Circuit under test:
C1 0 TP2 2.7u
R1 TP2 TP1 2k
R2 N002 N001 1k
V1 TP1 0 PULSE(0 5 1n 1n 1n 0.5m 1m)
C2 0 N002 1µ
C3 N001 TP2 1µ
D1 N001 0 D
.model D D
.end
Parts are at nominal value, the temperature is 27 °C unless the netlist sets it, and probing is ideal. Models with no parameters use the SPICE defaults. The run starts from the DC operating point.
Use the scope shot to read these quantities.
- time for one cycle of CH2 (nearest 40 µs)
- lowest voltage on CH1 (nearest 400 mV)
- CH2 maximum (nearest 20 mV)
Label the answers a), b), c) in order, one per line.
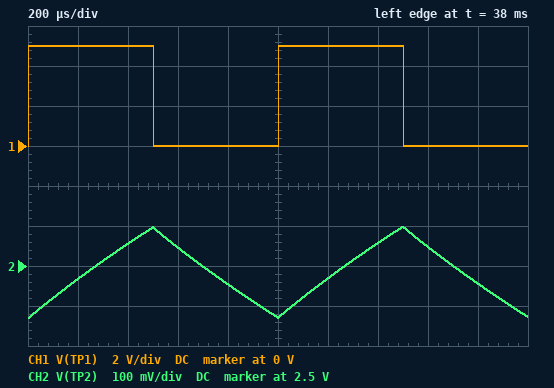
a) 1.00 ms
b) 0 V
c) 2.60 V
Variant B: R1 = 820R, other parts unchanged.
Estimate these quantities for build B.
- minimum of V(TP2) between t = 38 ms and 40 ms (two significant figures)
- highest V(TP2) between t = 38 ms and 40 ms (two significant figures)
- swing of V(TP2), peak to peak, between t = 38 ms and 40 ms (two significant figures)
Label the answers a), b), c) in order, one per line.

a) 2.2 V
b) 2.8 V
c) 550 mV
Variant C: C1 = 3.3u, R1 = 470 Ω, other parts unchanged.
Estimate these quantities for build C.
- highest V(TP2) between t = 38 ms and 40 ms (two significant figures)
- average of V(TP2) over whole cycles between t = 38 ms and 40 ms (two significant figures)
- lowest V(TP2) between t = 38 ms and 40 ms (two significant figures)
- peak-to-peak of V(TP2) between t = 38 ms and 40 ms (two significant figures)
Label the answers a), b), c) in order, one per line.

a) 2.9 V
b) 2.5 V
c) 2.1 V
d) 780 mV
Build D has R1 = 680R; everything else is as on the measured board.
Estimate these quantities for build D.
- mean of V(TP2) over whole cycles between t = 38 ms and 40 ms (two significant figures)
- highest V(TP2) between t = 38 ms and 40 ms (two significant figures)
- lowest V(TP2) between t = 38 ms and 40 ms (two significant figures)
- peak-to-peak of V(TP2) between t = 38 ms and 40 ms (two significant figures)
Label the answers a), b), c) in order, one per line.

a) 2.5 V
b) 2.8 V
c) 2.2 V
d) 660 mV
